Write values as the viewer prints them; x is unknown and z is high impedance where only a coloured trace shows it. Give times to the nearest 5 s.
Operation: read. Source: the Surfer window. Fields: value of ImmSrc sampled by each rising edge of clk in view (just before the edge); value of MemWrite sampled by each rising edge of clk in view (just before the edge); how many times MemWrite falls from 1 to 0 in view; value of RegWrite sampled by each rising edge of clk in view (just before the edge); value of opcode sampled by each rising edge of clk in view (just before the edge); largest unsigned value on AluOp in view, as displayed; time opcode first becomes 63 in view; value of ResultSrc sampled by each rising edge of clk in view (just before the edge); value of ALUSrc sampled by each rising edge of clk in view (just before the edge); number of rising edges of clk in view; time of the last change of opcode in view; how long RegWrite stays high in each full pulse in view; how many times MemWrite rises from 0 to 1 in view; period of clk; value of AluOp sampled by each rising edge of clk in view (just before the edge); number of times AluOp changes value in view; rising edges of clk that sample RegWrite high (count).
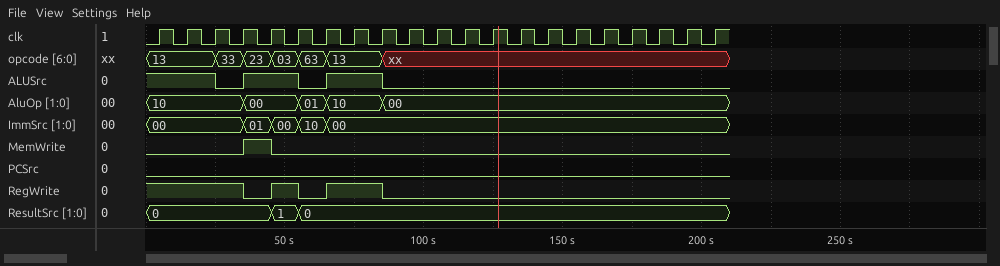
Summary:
00, 00, 00, 00, 01, 00, 10, 00, 00, 00, 00, 00, 00, 00, 00, 00, 00, 00, 00, 00, 00
0 0 0 0 1 0 0 0 0 0 0 0 0 0 0 0 0 0 0 0 0
1
1 1 1 1 0 1 0 1 1 0 0 0 0 0 0 0 0 0 0 0 0
13, 13, 13, 33, 23, 03, 63, 13, 13, xx, xx, xx, xx, xx, xx, xx, xx, xx, xx, xx, xx
10
55 s
0, 0, 0, 0, 0, 1, 0, 0, 0, 0, 0, 0, 0, 0, 0, 0, 0, 0, 0, 0, 0
1 1 1 0 1 1 0 1 1 0 0 0 0 0 0 0 0 0 0 0 0
21
85 s
10 s, 20 s
1
10 s
10, 10, 10, 10, 00, 00, 01, 10, 10, 00, 00, 00, 00, 00, 00, 00, 00, 00, 00, 00, 00
4
7
